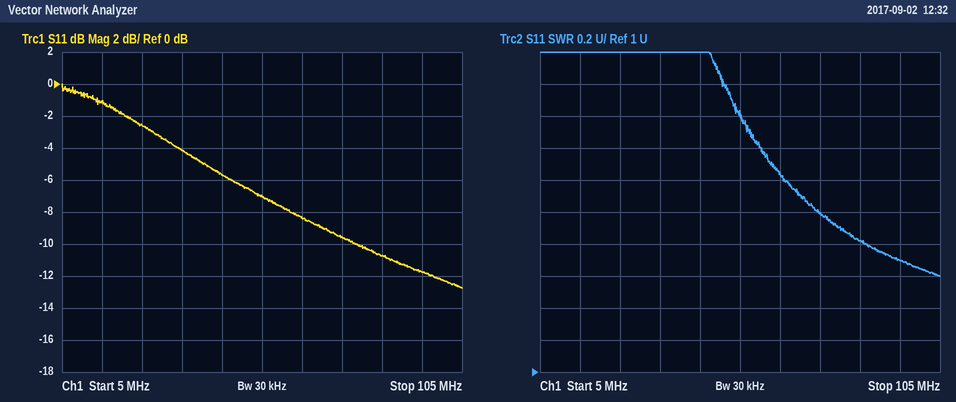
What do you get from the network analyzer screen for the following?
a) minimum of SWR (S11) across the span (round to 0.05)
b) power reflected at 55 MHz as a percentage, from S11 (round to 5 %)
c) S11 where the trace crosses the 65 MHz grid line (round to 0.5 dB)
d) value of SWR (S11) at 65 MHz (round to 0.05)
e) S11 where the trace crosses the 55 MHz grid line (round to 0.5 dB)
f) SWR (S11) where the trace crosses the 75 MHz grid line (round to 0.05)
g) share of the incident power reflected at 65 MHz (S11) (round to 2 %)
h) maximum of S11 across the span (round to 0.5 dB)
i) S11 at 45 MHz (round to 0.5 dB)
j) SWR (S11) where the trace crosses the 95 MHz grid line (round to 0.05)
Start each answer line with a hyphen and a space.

- 1.60
- 20 %
- -8.5 dB
- 2.25
- -7.0 dB
- 2.00
- 14 %
- 0.0 dB
- -5.5 dB
- 1.70
